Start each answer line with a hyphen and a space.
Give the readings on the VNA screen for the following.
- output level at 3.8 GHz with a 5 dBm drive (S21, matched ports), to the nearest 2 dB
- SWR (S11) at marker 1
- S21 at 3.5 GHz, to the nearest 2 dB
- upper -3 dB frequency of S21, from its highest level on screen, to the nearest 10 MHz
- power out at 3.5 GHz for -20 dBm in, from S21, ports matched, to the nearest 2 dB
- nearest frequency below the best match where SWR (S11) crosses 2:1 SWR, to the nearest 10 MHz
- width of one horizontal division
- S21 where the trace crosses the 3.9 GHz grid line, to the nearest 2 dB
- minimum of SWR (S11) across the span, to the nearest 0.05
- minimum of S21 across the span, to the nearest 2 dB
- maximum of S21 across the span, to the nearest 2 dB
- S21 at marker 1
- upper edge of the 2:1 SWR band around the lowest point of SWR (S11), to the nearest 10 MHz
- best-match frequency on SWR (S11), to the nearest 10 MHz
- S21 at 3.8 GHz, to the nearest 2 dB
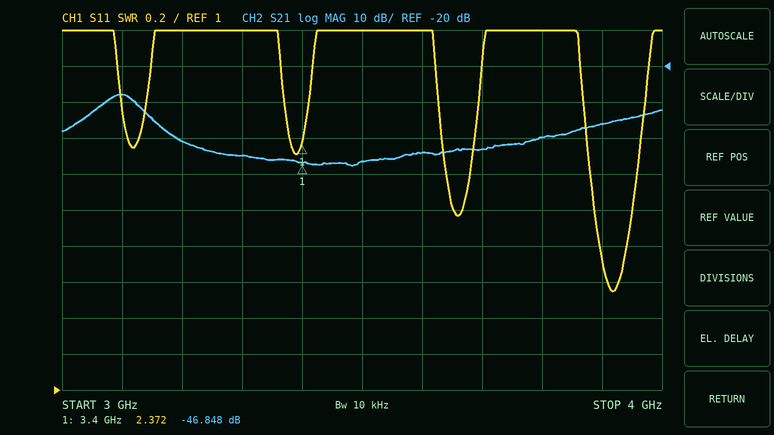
- -34 dBm
- 2.372
- -46 dB
- 3.13 GHz
- -66 dBm
- 3.89 GHz
- 100 MHz
- -36 dB
- 1.55
- -48 dB
- -28 dB
- -46.848 dB
- 3.95 GHz
- 3.92 GHz
- -40 dB
